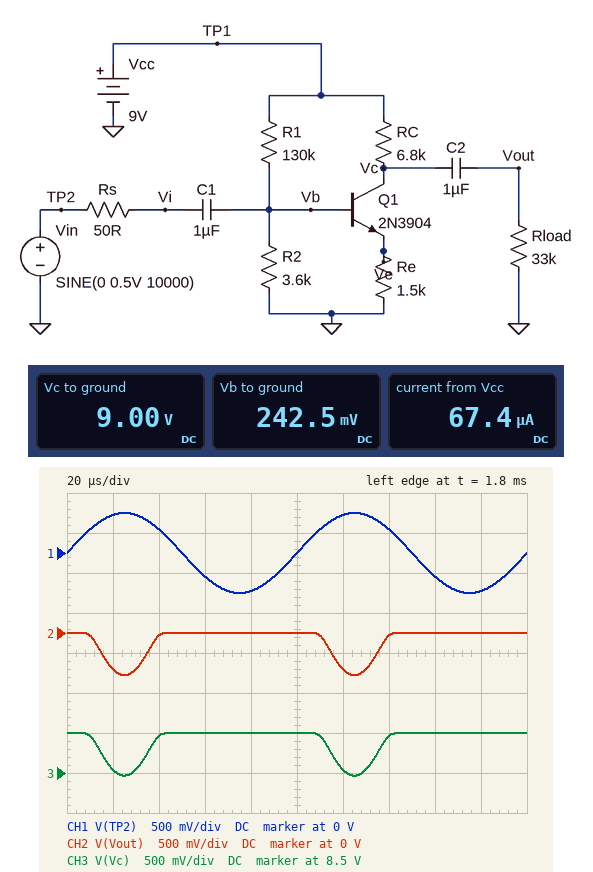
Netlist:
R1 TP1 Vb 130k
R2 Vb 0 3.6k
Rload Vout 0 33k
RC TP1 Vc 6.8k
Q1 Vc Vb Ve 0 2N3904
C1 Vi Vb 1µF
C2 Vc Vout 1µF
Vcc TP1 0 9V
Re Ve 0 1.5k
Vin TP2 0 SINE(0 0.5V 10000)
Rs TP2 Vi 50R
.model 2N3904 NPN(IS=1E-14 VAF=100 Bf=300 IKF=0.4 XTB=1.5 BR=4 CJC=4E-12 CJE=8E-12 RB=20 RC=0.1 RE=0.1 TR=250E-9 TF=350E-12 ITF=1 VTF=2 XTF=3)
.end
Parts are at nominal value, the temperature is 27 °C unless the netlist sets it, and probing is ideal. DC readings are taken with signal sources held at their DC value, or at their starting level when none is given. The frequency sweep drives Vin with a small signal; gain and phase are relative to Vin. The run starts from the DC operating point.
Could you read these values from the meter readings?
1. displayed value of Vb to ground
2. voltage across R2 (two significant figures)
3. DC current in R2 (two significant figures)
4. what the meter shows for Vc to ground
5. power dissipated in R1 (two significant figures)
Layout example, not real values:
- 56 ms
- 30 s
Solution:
- 242.5 mV
- 240 mV
- 67 µA
- 9.00 V
- 590 µW
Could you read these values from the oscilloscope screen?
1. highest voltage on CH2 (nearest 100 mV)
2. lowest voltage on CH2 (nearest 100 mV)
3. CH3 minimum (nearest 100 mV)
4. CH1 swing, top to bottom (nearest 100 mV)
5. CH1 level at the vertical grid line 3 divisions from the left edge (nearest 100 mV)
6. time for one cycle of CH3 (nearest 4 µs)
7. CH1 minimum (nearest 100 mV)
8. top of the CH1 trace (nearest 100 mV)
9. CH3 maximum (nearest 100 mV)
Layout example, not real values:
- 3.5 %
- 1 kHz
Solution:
- 0 V
- -500 mV
- 8.5 V
- 1.0 V
- -300 mV
- 100 µs
- -500 mV
- 500 mV
- 9.0 V
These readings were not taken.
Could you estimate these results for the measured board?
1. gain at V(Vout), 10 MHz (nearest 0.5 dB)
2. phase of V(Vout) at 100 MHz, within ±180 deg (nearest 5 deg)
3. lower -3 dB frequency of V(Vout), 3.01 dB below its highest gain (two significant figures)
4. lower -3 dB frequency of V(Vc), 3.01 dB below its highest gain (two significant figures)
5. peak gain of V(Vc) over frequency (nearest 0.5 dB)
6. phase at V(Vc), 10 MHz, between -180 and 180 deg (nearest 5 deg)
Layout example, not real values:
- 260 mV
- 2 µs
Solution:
- -6.0 dB
- 10 deg
- 16 MHz
- 16 MHz
- -0.5 dB
- 55 deg
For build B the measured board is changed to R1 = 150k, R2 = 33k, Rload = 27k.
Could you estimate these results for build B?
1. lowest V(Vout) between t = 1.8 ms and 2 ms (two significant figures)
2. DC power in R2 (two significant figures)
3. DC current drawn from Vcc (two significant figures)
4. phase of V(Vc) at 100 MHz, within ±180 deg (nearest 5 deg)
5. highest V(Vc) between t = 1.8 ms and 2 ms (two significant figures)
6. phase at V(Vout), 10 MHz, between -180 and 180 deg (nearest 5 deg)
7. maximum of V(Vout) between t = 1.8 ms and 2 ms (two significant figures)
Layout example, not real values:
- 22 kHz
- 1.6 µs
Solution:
- -1.8 V
- 75 µW
- 670 µA
- 25 deg
- 6.5 V
- 125 deg
- 1.7 V
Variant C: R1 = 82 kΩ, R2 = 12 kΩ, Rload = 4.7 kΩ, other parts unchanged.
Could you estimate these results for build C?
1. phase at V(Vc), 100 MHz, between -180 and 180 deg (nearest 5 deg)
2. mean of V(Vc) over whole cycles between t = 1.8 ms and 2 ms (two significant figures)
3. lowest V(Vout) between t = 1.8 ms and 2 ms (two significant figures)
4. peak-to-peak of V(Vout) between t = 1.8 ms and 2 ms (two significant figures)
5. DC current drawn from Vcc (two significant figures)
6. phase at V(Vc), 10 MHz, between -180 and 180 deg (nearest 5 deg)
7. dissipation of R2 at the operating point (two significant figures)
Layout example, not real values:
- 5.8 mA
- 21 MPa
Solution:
- 30 deg
- 6.7 V
- -880 mV
- 1.7 V
- 440 µA
- 145 deg
- 110 µW
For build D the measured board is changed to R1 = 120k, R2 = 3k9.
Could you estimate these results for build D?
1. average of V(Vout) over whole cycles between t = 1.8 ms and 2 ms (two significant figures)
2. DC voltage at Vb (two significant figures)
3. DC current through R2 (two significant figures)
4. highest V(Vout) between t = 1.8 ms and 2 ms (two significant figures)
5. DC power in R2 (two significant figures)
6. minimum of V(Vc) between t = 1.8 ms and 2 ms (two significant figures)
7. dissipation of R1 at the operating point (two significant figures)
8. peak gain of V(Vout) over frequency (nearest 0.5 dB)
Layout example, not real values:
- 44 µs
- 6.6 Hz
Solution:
- -130 mV
- 280 mV
- 73 µA
- 7.1 mV
- 21 µW
- 8.3 V
- 630 µW
- -0.5 dB
